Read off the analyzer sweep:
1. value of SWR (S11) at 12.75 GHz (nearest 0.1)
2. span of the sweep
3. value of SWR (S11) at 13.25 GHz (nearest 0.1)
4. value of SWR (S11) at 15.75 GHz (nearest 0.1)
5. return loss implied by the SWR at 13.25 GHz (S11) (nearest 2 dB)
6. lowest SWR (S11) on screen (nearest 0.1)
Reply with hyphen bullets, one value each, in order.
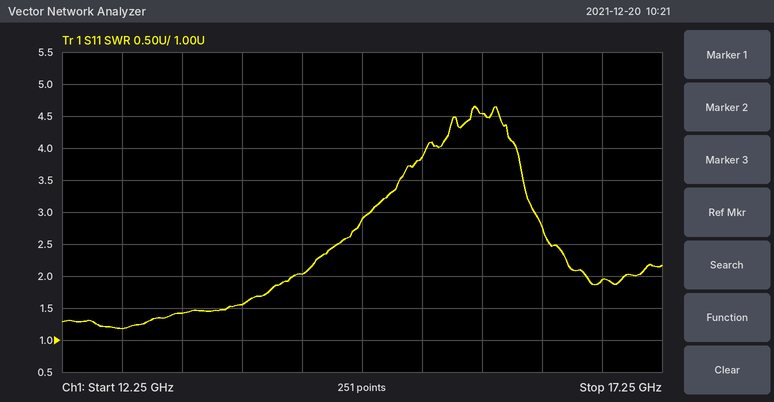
- 1.2
- 5 GHz
- 1.4
- 4.5
- 16 dB
- 1.2
